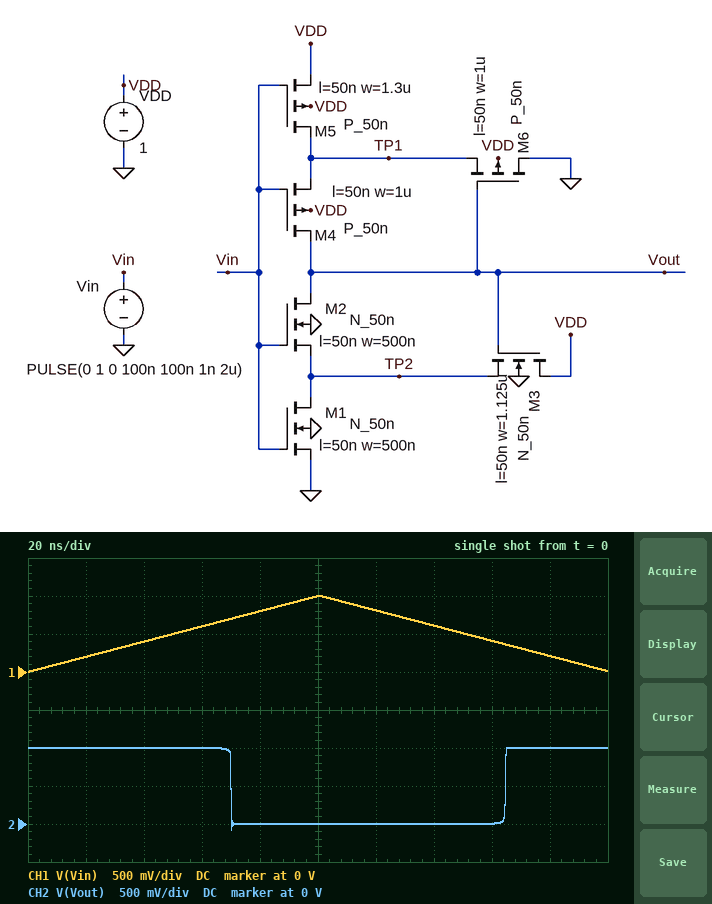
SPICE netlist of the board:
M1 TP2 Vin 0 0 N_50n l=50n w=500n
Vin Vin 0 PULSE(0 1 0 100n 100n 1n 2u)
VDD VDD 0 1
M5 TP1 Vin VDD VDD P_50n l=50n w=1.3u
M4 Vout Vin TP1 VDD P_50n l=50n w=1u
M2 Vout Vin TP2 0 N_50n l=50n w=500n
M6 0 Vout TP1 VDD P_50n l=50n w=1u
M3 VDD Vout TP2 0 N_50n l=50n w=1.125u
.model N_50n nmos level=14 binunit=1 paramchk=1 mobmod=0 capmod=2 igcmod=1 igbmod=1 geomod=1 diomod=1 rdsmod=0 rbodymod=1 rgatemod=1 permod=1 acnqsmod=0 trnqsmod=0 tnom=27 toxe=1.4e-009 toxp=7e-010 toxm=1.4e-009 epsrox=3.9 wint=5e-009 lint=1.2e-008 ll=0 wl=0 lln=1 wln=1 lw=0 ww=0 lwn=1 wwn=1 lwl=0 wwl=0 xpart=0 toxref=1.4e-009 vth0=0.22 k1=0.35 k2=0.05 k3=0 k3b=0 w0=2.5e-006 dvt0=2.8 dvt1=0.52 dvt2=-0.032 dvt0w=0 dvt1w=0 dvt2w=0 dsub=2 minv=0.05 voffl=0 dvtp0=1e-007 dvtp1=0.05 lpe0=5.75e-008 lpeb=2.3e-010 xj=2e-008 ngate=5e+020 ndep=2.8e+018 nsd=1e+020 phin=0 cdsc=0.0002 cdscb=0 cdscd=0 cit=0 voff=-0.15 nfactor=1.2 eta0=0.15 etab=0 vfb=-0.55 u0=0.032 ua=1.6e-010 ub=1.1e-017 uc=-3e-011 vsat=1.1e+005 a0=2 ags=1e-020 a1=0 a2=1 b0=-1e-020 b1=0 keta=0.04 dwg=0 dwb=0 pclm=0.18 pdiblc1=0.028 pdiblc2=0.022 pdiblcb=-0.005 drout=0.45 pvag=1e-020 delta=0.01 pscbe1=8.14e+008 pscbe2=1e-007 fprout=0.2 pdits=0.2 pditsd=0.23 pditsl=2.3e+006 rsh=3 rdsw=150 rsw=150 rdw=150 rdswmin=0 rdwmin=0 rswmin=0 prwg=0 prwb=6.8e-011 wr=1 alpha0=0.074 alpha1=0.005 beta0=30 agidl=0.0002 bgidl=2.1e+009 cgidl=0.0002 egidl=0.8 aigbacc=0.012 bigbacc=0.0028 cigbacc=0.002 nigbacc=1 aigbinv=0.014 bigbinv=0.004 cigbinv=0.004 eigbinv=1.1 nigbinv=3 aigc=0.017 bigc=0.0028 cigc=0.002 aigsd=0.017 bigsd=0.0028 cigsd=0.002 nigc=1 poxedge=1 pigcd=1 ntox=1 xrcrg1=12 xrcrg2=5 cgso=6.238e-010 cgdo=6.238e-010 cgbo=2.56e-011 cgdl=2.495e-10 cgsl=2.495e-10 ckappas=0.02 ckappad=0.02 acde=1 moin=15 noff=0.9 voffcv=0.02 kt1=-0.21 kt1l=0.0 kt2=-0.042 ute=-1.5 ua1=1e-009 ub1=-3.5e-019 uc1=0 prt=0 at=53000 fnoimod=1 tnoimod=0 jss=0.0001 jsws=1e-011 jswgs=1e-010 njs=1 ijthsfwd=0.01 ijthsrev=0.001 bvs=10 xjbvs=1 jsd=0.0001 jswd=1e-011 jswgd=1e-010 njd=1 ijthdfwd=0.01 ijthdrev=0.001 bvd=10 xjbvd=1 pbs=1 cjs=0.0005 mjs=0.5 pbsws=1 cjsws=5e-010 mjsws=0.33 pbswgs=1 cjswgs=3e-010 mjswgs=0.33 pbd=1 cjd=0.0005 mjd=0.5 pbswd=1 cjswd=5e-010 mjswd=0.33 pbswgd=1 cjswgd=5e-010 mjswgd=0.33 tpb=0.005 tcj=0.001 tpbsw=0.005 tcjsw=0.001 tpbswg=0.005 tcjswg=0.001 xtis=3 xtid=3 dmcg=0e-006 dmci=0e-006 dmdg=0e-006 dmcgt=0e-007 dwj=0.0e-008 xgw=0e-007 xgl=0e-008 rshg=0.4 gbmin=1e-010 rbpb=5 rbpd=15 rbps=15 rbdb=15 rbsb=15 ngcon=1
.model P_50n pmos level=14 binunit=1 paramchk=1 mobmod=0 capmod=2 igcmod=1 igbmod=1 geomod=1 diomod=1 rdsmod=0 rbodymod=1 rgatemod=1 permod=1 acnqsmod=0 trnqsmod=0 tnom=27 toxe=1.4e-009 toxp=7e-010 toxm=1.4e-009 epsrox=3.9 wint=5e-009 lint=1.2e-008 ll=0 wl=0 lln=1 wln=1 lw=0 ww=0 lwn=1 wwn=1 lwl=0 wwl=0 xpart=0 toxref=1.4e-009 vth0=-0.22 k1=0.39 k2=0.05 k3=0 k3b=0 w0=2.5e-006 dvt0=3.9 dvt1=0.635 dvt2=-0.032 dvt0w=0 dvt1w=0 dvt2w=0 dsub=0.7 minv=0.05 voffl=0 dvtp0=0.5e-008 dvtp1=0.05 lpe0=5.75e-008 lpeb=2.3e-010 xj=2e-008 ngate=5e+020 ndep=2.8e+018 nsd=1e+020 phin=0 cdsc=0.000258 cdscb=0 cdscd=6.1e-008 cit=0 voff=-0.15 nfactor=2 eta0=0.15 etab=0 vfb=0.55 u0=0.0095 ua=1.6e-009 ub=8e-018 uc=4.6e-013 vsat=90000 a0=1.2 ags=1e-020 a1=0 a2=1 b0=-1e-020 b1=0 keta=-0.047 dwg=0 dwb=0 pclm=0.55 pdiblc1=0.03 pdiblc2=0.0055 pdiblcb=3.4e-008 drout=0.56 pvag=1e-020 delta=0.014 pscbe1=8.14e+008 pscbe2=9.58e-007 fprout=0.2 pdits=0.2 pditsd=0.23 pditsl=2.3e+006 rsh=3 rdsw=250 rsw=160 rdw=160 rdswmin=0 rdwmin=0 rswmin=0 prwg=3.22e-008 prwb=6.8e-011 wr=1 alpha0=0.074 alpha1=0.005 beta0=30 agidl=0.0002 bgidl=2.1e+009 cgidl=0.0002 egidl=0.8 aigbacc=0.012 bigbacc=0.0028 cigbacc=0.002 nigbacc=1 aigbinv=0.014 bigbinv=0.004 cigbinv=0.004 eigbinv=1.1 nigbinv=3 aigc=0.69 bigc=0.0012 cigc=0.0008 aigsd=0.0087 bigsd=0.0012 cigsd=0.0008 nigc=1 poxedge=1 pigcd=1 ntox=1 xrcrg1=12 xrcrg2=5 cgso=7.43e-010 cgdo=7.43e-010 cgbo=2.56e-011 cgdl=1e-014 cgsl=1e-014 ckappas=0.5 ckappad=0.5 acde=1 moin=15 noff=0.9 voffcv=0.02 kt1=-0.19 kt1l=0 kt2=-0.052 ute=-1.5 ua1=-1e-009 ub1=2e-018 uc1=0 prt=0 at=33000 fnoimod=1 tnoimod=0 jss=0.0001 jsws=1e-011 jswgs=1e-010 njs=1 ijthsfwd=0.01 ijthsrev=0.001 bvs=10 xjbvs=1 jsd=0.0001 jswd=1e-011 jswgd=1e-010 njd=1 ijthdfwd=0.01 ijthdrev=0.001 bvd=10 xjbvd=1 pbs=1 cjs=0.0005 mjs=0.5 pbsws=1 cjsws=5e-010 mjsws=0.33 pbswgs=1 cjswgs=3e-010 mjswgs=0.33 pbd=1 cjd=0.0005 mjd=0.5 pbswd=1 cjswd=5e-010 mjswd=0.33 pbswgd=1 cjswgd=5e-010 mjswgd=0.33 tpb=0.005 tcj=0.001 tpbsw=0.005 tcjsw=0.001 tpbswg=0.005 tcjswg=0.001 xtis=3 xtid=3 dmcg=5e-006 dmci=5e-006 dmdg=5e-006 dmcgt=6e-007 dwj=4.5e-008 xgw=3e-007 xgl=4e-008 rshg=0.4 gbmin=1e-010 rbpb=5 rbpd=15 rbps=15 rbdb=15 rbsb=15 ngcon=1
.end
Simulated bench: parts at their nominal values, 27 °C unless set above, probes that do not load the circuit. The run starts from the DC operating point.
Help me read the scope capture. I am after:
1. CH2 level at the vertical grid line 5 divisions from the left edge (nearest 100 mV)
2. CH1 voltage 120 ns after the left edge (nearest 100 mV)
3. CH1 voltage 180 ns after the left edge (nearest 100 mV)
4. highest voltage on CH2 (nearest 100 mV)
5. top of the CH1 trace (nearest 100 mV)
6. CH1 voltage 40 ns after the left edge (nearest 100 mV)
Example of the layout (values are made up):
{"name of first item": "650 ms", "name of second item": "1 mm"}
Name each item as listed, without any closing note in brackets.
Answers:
{"CH2 level at the vertical grid line 5 divisions from the left edge": "0 V", "CH1 voltage 120 ns after the left edge": "800 mV", "CH1 voltage 180 ns after the left edge": "200 mV", "highest voltage on CH2": "1.0 V", "top of the CH1 trace": "1.0 V", "CH1 voltage 40 ns after the left edge": "400 mV"}
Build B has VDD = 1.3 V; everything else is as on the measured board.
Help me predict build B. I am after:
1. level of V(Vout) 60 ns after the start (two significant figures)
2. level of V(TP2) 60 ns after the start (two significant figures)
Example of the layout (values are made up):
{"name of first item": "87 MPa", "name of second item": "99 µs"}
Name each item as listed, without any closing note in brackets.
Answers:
{"level of V(Vout) 60 ns after the start": "1.3 V", "level of V(TP2) 60 ns after the start": "750 mV"}
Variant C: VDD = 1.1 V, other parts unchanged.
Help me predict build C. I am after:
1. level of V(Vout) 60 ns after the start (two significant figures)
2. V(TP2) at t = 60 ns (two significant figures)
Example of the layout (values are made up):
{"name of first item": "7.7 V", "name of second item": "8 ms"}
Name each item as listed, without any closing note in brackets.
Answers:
{"level of V(Vout) 60 ns after the start": "1.1 V", "V(TP2) at t = 60 ns": "570 mV"}
